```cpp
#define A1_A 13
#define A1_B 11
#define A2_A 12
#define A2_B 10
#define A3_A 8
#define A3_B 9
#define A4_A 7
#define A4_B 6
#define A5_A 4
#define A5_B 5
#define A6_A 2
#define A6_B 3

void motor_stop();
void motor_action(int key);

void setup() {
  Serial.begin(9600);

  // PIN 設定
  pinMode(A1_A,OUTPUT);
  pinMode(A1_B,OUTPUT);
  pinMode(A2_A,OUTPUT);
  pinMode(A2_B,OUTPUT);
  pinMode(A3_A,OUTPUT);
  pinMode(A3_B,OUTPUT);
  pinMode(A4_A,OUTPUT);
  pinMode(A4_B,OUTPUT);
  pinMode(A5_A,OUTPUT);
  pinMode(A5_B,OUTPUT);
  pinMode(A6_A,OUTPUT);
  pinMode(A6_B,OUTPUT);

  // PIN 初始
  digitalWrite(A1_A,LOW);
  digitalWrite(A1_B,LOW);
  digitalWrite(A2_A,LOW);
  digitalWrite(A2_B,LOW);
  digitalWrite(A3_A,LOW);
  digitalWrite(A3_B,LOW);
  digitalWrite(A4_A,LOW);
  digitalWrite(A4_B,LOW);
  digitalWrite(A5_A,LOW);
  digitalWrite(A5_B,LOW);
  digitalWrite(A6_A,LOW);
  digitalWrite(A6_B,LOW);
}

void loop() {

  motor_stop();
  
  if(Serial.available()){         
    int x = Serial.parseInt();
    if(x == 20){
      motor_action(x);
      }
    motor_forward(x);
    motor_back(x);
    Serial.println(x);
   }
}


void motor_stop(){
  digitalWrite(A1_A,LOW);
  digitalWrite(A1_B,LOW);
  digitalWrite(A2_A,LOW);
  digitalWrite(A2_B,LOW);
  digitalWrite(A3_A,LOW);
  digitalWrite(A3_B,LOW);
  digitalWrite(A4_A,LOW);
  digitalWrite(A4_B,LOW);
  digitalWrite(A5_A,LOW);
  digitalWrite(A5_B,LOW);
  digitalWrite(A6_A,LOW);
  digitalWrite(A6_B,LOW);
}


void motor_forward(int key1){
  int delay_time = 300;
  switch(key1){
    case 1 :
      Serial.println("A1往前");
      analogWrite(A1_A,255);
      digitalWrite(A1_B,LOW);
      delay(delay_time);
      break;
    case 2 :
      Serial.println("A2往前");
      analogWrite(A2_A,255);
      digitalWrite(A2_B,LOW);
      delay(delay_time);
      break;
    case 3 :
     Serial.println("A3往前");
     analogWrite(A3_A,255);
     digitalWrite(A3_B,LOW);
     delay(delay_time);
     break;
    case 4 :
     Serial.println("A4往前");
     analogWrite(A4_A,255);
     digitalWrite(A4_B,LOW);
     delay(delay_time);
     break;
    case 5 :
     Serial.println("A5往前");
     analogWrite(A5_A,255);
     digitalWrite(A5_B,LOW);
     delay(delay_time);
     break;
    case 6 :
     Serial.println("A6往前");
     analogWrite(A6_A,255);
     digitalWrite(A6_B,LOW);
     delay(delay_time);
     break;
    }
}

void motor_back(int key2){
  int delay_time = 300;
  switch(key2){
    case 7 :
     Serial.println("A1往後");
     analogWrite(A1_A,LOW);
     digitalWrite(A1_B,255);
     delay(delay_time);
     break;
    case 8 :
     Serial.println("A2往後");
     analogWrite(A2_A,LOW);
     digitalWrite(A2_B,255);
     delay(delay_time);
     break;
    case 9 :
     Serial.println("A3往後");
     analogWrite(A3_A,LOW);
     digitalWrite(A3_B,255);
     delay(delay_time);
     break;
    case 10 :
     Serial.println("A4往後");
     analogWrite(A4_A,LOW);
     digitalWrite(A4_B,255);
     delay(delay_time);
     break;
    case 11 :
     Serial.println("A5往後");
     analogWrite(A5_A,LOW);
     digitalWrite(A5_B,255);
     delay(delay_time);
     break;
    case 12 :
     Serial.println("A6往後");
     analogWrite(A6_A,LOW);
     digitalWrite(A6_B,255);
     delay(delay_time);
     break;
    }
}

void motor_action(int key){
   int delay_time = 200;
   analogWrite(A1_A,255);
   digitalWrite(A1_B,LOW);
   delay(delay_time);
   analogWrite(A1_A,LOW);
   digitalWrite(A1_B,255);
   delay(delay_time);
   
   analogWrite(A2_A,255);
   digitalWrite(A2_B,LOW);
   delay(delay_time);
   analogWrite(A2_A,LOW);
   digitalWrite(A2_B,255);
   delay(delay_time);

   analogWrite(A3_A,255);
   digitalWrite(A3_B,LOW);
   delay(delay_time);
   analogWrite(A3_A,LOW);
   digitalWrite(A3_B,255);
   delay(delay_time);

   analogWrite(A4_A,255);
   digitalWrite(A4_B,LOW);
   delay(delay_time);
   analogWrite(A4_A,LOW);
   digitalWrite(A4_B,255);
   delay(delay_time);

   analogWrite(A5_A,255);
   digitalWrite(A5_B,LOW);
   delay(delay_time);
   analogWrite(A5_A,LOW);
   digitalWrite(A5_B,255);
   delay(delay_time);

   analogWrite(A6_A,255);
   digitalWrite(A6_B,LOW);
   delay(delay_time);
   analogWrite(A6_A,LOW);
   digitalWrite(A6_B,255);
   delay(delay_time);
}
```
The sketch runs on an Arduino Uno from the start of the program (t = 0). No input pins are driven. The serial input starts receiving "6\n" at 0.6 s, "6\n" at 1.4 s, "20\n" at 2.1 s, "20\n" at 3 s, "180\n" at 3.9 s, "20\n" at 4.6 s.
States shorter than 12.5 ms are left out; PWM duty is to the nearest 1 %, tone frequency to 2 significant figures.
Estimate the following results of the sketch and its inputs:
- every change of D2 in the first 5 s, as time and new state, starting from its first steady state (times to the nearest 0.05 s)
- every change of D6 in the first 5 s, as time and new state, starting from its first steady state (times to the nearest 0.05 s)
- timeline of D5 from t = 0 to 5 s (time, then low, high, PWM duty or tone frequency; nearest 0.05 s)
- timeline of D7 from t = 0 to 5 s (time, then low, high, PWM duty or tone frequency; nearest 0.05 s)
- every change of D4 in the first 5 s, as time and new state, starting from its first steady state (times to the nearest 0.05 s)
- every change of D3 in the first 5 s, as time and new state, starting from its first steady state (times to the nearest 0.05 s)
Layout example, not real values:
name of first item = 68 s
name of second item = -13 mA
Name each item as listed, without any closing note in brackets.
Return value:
every change of D2 in the first 5 s, as time and new state, starting from its first steady state = 0 s low; 0.6 s high; 0.9 s low; 1.4 s high; 1.7 s low; 4.1 s high; 4.3 s low
every change of D6 in the first 5 s, as time and new state, starting from its first steady state = 0 s low; 3.5 s high; 4.5 s low
timeline of D5 from t = 0 to 5 s = 0 s low; 3.9 s high; 4.5 s low
timeline of D7 from t = 0 to 5 s = 0 s low; 3.3 s high; 3.5 s low
every change of D4 in the first 5 s, as time and new state, starting from its first steady state = 0 s low; 3.7 s high; 3.9 s low
every change of D3 in the first 5 s, as time and new state, starting from its first steady state = 0 s low; 4.3 s high; 4.5 s low
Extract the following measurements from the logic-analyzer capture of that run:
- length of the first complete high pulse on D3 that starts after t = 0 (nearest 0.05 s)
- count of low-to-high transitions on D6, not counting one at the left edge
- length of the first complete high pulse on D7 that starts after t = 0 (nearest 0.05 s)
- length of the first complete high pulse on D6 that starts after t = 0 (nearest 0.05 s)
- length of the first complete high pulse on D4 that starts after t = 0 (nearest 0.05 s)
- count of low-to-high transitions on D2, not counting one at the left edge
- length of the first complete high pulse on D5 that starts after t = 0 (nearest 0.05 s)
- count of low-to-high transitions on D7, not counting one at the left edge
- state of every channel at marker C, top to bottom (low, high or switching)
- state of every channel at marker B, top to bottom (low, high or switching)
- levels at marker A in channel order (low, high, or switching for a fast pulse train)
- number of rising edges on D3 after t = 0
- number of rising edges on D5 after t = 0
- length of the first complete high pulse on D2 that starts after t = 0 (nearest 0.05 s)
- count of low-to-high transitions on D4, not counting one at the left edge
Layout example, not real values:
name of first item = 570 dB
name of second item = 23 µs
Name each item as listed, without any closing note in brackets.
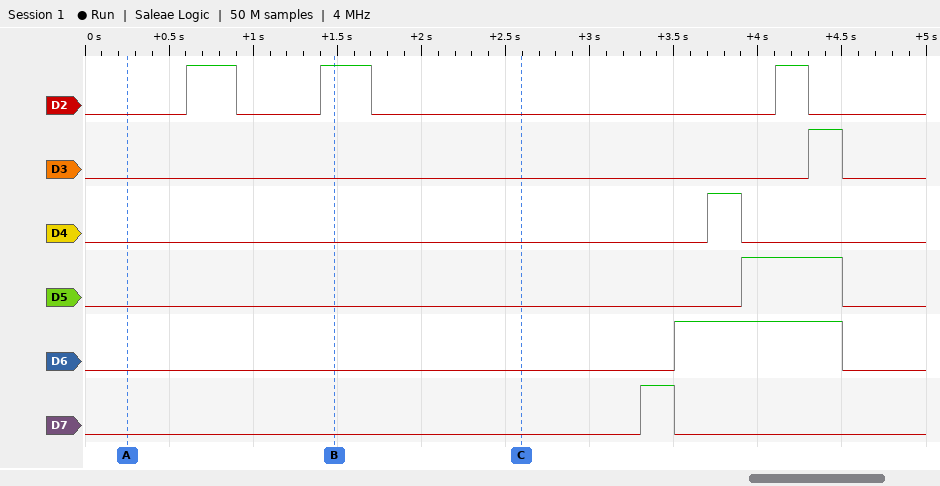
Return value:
length of the first complete high pulse on D3 that starts after t = 0 = 0.20 s
count of low-to-high transitions on D6, not counting one at the left edge = 1
length of the first complete high pulse on D7 that starts after t = 0 = 0.20 s
length of the first complete high pulse on D6 that starts after t = 0 = 1.00 s
length of the first complete high pulse on D4 that starts after t = 0 = 0.20 s
count of low-to-high transitions on D2, not counting one at the left edge = 3
length of the first complete high pulse on D5 that starts after t = 0 = 0.60 s
count of low-to-high transitions on D7, not counting one at the left edge = 1
state of every channel at marker C, top to bottom = D2 low, D3 low, D4 low, D5 low, D6 low, D7 low
state of every channel at marker B, top to bottom = D2 high, D3 low, D4 low, D5 low, D6 low, D7 low
levels at marker A in channel order = D2 low, D3 low, D4 low, D5 low, D6 low, D7 low
number of rising edges on D3 after t = 0 = 1
number of rising edges on D5 after t = 0 = 1
length of the first complete high pulse on D2 that starts after t = 0 = 0.30 s
count of low-to-high transitions on D4, not counting one at the left edge = 1
